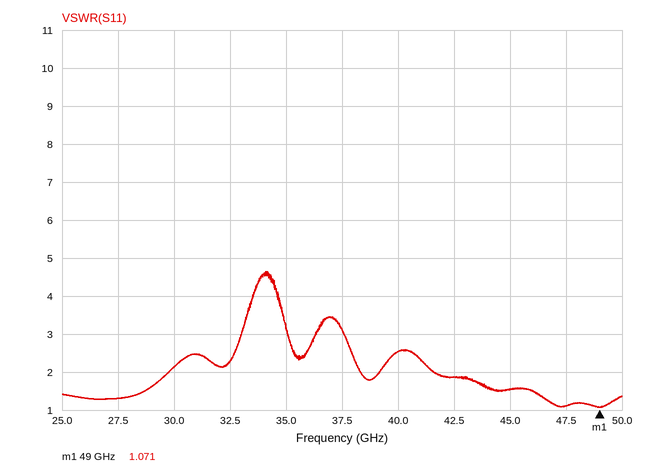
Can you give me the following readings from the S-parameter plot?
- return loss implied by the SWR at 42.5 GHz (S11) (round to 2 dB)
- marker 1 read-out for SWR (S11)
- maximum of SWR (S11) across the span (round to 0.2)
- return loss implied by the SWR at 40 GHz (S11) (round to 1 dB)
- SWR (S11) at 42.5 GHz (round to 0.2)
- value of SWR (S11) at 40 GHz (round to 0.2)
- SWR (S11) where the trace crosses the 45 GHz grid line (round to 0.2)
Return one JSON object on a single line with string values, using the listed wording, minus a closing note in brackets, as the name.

{"return loss implied by the SWR at 42.5 GHz (S11)": "10 dB", "marker 1 read-out for SWR": "1.071", "maximum of SWR (S11) across the span": "4.6", "return loss implied by the SWR at 40 GHz (S11)": "7 dB", "SWR (S11) at 42.5 GHz": "1.8", "value of SWR (S11) at 40 GHz": "2.6", "SWR (S11) where the trace crosses the 45 GHz grid line": "1.6"}
